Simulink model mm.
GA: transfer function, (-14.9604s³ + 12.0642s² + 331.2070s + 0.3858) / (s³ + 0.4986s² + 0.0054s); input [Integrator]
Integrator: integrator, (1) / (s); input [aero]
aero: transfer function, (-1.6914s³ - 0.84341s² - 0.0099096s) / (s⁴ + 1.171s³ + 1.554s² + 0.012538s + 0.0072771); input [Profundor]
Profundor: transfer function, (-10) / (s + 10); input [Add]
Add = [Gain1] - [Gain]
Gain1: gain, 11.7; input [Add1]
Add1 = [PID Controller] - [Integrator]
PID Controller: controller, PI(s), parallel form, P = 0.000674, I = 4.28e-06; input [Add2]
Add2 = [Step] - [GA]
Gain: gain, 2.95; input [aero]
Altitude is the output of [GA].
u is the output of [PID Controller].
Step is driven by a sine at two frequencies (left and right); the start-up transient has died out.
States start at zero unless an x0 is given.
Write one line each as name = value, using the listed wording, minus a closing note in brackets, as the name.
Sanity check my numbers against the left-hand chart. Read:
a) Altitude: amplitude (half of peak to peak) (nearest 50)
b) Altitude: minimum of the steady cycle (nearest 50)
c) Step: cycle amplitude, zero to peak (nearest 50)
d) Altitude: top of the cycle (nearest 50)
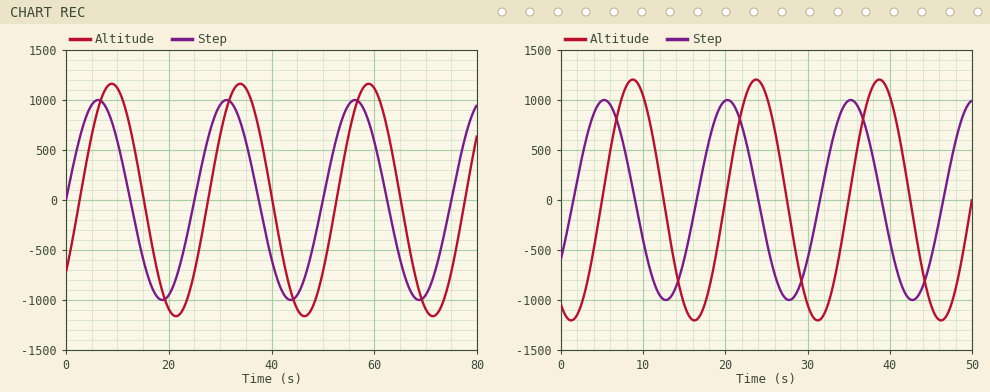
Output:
Altitude: amplitude (half of peak to peak) = 1150
Altitude: minimum of the steady cycle = -1150
Step: cycle amplitude, zero to peak = 1000
Altitude: top of the cycle = 1150
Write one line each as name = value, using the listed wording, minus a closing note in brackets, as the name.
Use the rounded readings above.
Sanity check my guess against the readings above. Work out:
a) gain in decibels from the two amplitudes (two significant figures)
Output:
gain in decibels from the two amplitudes = 1.2 dB
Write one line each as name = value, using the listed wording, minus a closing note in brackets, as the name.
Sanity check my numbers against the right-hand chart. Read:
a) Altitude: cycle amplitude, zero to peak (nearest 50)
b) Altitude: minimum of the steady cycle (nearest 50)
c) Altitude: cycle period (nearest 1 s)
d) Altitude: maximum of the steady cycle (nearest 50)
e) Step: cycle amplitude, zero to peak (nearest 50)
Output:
Altitude: cycle amplitude, zero to peak = 1200
Altitude: minimum of the steady cycle = -1200
Altitude: cycle period = 15 s
Altitude: maximum of the steady cycle = 1200
Step: cycle amplitude, zero to peak = 1000
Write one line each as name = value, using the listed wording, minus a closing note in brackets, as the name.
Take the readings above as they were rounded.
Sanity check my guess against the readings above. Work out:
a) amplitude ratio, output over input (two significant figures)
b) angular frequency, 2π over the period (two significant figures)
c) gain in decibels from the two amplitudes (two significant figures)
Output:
amplitude ratio, output over input = 1.2
angular frequency, 2π over the period = 0.42 rad/s
gain in decibels from the two amplitudes = 1.6 dB
